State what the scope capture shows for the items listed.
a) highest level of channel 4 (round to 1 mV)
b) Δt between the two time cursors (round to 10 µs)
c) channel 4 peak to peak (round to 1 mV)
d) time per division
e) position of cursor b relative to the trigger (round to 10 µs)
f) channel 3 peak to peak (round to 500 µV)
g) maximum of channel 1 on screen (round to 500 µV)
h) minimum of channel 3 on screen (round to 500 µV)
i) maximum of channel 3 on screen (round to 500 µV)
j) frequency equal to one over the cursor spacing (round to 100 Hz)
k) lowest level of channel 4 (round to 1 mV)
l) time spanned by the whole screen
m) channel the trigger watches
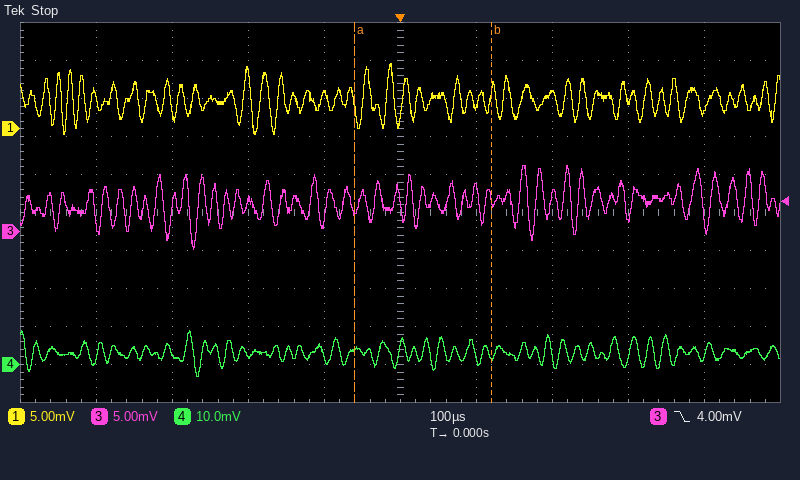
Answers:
9 mV
180 µs
12 mV
100 µs
+120 µs
11.0 mV
8.5 mV
-2.5 mV
8.5 mV
5.6 kHz
-3 mV
1 ms
channel 3
